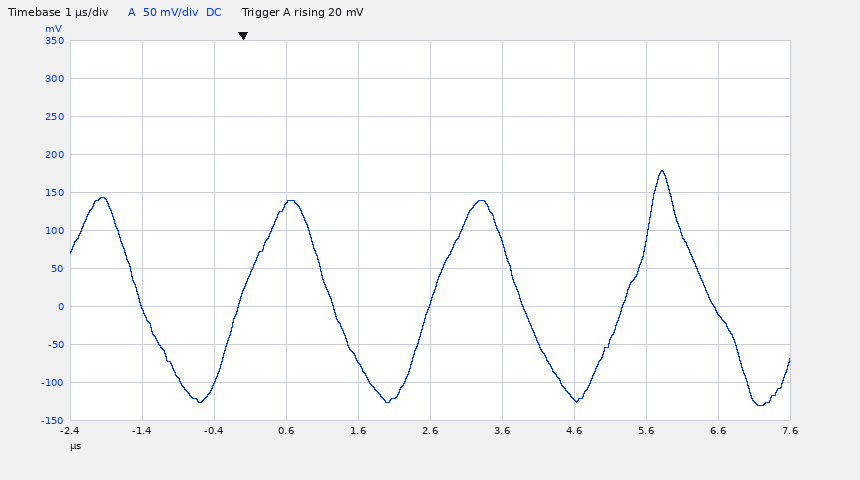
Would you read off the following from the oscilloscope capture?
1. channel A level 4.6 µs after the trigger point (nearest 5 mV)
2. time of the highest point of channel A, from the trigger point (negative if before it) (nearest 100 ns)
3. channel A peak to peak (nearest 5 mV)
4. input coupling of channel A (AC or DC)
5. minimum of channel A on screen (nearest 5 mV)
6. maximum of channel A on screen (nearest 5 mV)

-120 mV
+5.8 µs
310 mV
DC
-130 mV
180 mV
